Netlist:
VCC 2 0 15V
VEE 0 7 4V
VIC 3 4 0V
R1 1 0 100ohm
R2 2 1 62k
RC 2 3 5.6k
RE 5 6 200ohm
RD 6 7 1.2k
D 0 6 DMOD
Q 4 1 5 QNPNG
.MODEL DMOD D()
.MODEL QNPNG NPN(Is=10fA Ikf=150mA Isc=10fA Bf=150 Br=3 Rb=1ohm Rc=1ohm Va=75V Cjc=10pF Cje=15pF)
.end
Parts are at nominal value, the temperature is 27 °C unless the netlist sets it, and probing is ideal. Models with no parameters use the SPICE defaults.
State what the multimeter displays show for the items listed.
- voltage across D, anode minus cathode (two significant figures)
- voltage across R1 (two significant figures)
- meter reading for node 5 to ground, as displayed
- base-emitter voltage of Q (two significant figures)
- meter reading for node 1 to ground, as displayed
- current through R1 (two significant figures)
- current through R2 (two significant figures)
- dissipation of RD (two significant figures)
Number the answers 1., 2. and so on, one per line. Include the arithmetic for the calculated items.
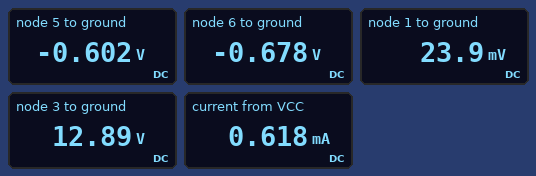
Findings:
1. 0 V - (-678 mV) = 680 mV
2. 23.9 mV = 24 mV
3. -0.602 V
4. 23.9 mV - (-602 mV) = 630 mV
5. 23.9 mV
6. (23.9 mV) / 100 Ω = 240 µA
7. (15 V - 23.9 mV) / 62 kΩ = 240 µA
8. (-678 mV - (-4 V))^2 / 1.2 kΩ = 9.2 mW
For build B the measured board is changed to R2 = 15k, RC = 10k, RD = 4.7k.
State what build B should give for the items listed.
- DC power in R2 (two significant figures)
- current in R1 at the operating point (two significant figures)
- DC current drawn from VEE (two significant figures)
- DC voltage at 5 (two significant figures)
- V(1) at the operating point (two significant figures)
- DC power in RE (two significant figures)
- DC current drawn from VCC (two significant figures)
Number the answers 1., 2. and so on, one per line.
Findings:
1. 15 mW
2. 990 µA
3. 720 µA
4. -530 mV
5. 99 mV
6. 40 µW
7. 1.4 mA
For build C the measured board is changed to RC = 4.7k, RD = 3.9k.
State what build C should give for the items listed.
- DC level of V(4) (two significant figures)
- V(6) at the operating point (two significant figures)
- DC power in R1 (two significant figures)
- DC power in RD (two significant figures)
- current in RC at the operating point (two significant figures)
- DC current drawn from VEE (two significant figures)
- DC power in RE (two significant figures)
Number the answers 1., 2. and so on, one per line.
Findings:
1. 14 V
2. -640 mV
3. 5.8 µW
4. 2.9 mW
5. 250 µA
6. 860 µA
7. 13 µW
